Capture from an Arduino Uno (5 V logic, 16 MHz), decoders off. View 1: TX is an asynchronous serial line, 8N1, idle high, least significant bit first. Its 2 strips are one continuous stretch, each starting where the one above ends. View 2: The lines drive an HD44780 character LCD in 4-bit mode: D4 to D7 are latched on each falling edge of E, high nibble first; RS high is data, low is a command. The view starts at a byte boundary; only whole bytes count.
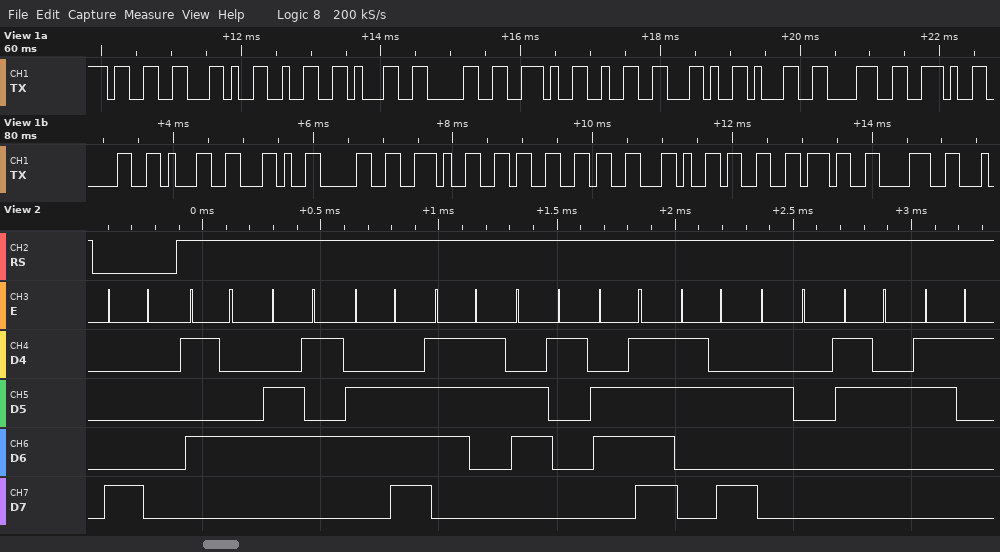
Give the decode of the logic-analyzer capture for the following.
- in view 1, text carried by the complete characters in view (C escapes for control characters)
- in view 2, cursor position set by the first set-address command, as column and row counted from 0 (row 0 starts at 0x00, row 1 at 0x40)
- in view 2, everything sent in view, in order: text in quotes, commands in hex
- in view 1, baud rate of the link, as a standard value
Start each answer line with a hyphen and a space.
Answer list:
- "3,210.2,18.01,0.66,378"
- column 0, row 0
- 0x80 "Tensao: 21"
- 9600 baud
